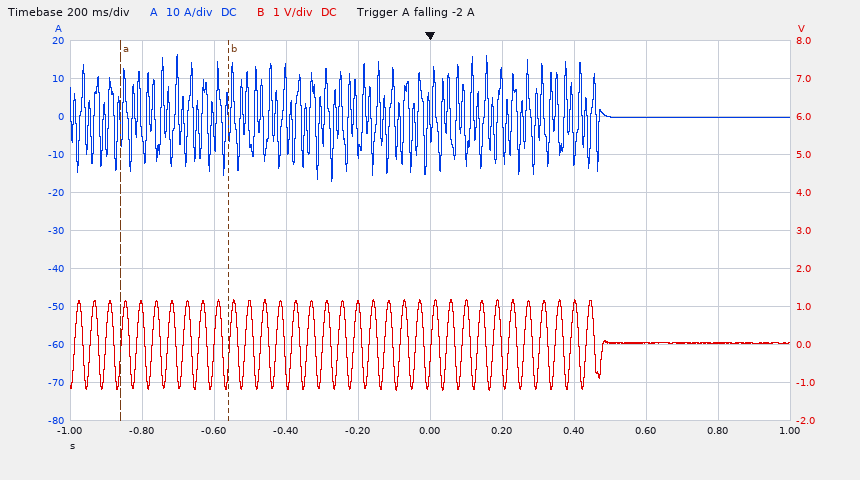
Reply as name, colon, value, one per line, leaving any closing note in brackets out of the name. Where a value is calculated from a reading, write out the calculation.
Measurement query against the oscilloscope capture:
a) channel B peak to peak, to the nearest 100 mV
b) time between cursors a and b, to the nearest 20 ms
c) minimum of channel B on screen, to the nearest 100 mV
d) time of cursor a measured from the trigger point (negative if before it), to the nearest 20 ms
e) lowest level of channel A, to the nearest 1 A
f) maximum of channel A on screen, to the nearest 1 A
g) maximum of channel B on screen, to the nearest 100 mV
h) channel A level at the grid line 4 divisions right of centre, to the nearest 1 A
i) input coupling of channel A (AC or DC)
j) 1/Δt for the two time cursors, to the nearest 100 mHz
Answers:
channel B peak to peak, to the nearest 100 mV: 1.2 V − (-1.2 V) = 2.4 V
time between cursors a and b, to the nearest 20 ms: 300 ms
minimum of channel B on screen, to the nearest 100 mV: -1.2 V
time of cursor a measured from the trigger point (negative if before it), to the nearest 20 ms: -860 ms
lowest level of channel A, to the nearest 1 A: -17 A
maximum of channel A on screen, to the nearest 1 A: 16 A
maximum of channel B on screen, to the nearest 100 mV: 1.2 V
channel A level at the grid line 4 divisions right of centre, to the nearest 1 A: 0 A
input coupling of channel A: DC
1/Δt for the two time cursors, to the nearest 100 mHz: 1 / 300 ms ≈ 3.3 Hz
